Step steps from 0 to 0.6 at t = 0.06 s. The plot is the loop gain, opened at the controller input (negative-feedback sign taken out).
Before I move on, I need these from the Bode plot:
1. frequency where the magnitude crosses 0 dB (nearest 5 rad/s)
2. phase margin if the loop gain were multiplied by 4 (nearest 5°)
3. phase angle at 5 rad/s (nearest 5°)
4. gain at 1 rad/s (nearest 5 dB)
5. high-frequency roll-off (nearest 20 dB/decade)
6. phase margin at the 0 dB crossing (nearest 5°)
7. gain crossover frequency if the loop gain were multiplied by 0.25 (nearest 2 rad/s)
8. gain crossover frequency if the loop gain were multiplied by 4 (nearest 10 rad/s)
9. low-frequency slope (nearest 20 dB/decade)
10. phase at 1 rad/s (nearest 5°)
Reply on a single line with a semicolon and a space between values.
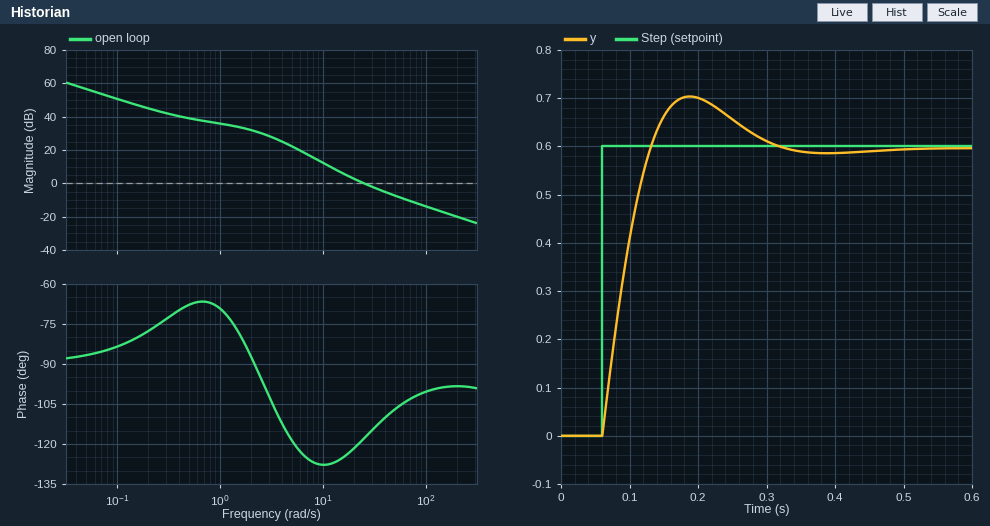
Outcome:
25 rad/s; 80°; -120°; 35 dB; -20 dB/decade; 60°; 10 rad/s; 80 rad/s; -20 dB/decade; -70°
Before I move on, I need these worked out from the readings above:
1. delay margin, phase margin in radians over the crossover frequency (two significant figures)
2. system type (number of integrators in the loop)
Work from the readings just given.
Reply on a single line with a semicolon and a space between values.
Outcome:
0.042 s; 1
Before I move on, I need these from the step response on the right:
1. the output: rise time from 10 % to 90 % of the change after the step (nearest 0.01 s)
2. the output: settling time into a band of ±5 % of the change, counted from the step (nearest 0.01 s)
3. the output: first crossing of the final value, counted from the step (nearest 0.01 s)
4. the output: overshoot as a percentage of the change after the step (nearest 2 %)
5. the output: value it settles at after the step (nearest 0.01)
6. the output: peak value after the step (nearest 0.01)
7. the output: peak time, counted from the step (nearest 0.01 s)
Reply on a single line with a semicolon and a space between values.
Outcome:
0.05 s; 0.22 s; 0.07 s; 18 %; 0.60; 0.70; 0.13 s
